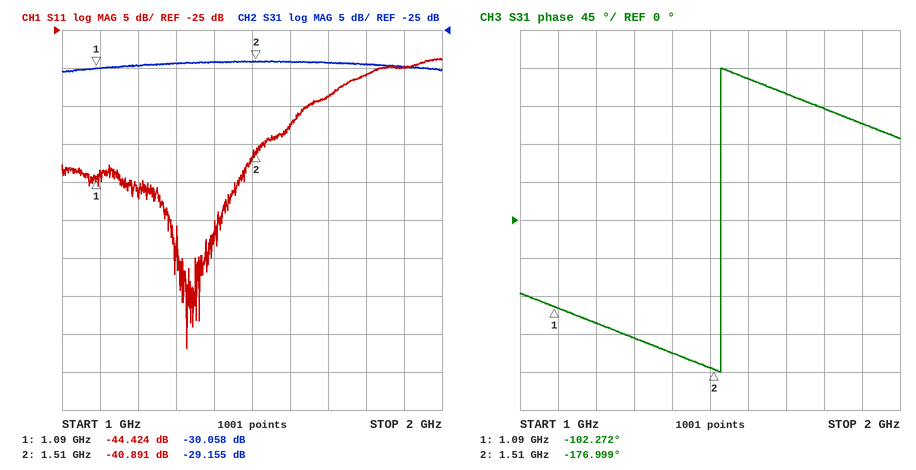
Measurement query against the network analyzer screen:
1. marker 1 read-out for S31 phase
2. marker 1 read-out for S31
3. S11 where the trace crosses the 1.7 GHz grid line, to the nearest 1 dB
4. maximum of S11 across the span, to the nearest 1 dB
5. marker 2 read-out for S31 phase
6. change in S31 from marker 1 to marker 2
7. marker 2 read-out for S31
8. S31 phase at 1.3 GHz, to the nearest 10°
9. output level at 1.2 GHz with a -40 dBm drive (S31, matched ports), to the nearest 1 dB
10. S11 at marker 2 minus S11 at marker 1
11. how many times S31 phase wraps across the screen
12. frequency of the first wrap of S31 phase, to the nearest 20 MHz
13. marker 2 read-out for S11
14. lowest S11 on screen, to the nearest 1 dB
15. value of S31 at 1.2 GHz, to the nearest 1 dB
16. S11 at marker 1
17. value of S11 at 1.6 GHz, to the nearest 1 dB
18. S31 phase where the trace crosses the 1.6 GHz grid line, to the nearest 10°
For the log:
-102.272°
-30.058 dB
-34 dB
-29 dB
-176.999°
0.903 dB
-29.155 dB
-140°
-70 dBm
3.533 dB
1
1.52 GHz
-40.891 dB
-67 dB
-30 dB
-44.424 dB
-38 dB
170°
